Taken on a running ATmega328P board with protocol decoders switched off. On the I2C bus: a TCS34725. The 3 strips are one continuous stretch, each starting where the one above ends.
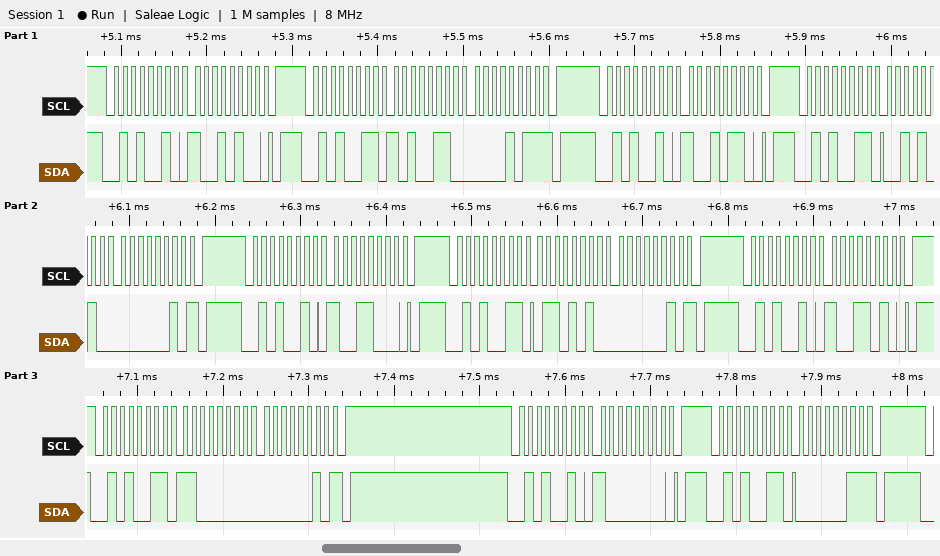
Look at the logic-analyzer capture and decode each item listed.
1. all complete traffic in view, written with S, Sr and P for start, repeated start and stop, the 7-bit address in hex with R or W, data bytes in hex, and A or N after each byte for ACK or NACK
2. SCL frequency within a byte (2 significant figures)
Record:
S 29W A 94 A P S 29R A A6 A 0B N P S 29W A 96 A P S 29R A 2A A 02 N P S 29W A 98 A P S 29R A 6A A 02 N P S 29W A 9A A P S 29R A C0 A 02 N P S 29W A 80 A P S 29R A 03 N P
100 kHz
